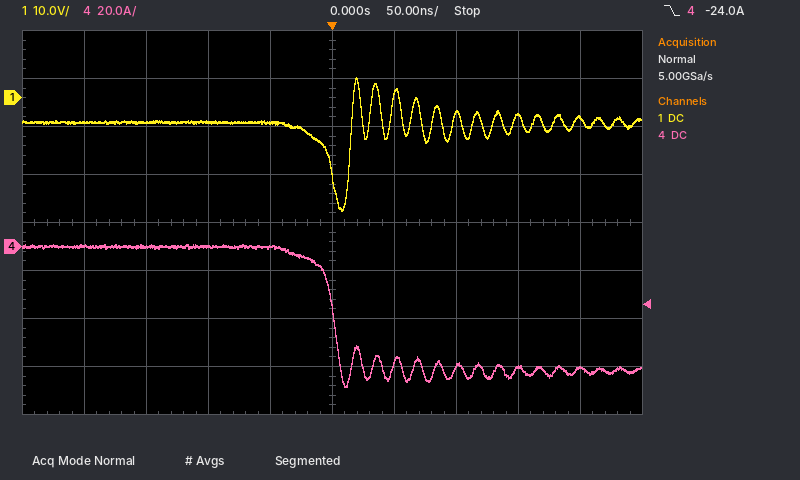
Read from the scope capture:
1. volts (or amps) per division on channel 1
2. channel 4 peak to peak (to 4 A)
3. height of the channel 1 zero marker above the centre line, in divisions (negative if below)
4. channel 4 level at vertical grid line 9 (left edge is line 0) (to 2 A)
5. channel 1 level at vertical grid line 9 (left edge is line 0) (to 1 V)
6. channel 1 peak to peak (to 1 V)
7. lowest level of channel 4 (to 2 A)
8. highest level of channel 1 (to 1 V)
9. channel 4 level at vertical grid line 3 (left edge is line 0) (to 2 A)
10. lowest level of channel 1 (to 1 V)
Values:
10 V
60 A
+2.6 div
-50 A
-4 V
28 V
-58 A
4 V
0 A
-24 V
